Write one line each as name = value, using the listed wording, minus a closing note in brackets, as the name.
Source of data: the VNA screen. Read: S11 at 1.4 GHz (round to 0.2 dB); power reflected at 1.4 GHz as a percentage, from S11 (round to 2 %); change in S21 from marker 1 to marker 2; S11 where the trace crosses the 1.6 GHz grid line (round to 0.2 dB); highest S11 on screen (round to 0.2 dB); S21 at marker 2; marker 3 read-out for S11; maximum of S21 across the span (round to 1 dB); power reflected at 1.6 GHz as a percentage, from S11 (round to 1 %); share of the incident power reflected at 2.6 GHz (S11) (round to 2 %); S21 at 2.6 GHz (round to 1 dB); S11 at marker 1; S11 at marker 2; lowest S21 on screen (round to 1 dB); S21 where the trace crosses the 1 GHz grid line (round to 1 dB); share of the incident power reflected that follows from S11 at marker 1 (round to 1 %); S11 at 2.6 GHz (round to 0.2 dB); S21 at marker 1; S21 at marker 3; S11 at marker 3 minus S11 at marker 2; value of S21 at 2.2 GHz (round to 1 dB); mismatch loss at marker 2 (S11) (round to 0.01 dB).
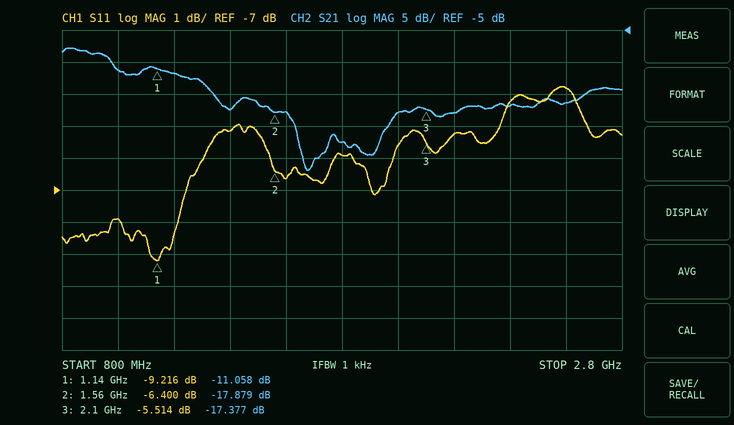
S11 at 1.4 GHz = -5.2 dB
power reflected at 1.4 GHz as a percentage, from S11 = 30 %
change in S21 from marker 1 to marker 2 = -6.821 dB
S11 where the trace crosses the 1.6 GHz grid line = -6.6 dB
highest S11 on screen = -3.8 dB
S21 at marker 2 = -17.879 dB
marker 3 read-out for S11 = -5.514 dB
maximum of S21 across the span = -8 dB
power reflected at 1.6 GHz as a percentage, from S11 = 22 %
share of the incident power reflected at 2.6 GHz (S11) = 42 %
S21 at 2.6 GHz = -16 dB
S11 at marker 1 = -9.216 dB
S11 at marker 2 = -6.400 dB
lowest S21 on screen = -27 dB
S21 where the trace crosses the 1 GHz grid line = -11 dB
share of the incident power reflected that follows from S11 at marker 1 = 12 %
S11 at 2.6 GHz = -3.8 dB
S21 at marker 1 = -11.058 dB
S21 at marker 3 = -17.377 dB
S11 at marker 3 minus S11 at marker 2 = 0.886 dB
value of S21 at 2.2 GHz = -18 dB
mismatch loss at marker 2 (S11) = 1.13 dB
